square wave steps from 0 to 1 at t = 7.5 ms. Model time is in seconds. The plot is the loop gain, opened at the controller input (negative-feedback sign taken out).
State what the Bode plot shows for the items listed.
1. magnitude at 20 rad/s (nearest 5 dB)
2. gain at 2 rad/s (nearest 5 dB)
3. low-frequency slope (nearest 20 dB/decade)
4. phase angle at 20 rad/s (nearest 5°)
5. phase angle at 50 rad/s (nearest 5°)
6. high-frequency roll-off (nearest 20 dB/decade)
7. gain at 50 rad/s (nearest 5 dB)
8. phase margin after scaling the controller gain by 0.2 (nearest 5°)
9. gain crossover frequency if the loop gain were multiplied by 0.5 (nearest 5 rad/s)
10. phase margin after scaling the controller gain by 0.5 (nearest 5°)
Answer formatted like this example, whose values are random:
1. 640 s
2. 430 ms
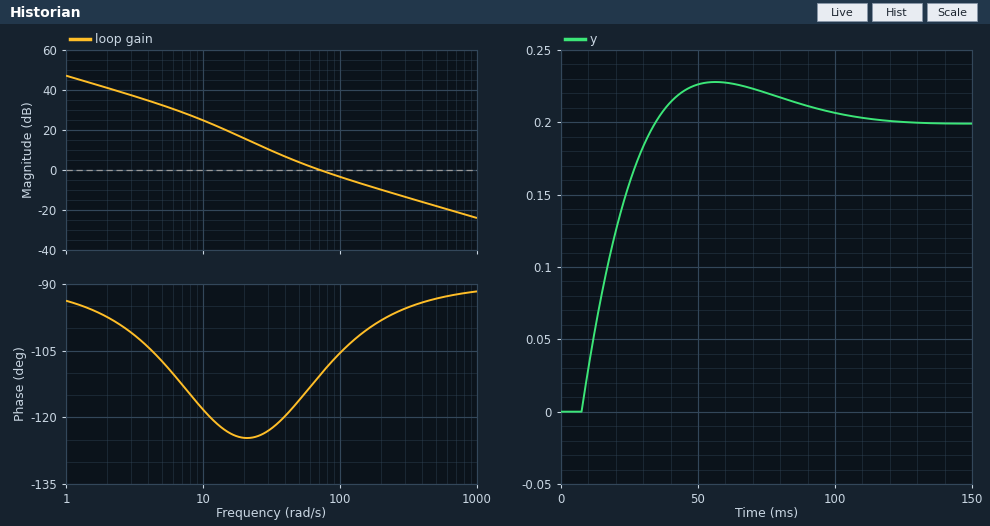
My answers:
1. 15 dB
2. 40 dB
3. -20 dB/decade
4. -125°
5. -115°
6. -20 dB/decade
7. 5 dB
8. 55°
9. 40 rad/s
10. 60°
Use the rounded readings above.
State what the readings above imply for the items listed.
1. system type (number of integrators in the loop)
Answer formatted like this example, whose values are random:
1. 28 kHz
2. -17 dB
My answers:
1. 1
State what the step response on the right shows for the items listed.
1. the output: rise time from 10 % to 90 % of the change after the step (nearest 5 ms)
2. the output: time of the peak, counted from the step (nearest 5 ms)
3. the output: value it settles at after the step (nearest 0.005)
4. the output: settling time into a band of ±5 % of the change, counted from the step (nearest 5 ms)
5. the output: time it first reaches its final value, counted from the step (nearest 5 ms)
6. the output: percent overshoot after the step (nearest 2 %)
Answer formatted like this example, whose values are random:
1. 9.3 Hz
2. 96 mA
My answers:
1. 20 ms
2. 50 ms
3. 0.200
4. 85 ms
5. 25 ms
6. 14 %
